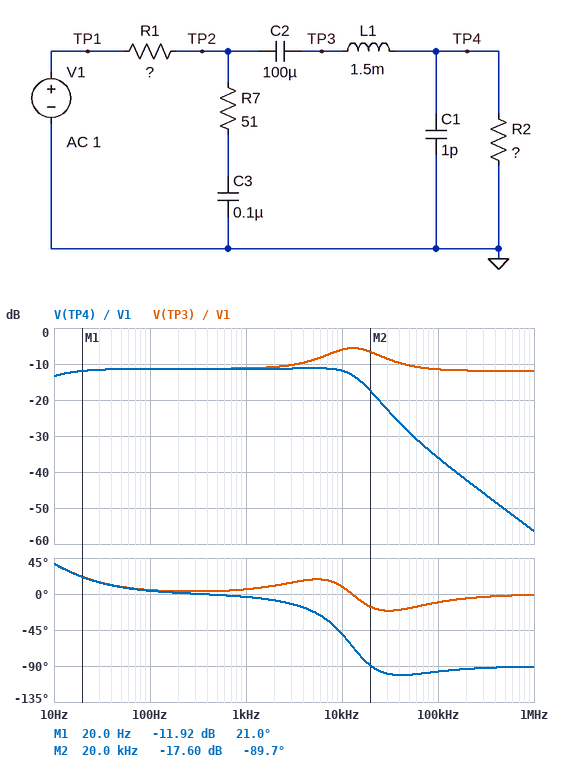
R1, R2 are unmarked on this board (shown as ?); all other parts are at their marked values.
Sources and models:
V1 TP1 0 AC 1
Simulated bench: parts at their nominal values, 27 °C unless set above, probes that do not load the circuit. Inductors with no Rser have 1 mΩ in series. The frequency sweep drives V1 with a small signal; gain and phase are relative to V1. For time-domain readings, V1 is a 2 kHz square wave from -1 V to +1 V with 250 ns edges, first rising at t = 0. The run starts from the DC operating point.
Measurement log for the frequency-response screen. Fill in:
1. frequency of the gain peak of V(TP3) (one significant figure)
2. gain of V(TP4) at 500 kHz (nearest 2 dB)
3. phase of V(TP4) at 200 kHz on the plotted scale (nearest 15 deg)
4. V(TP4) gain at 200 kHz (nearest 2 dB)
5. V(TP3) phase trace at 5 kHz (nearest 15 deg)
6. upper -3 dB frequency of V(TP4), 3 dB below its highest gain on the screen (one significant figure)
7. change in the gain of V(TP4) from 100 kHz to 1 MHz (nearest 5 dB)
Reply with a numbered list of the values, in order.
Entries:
1. 10 kHz
2. -50 dB
3. -90 deg
4. -42 dB
5. 15 deg
6. 10 kHz
7. -20 dB
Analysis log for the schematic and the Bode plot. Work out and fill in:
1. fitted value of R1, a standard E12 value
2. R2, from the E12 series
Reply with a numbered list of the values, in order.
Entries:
1. 150 Ω
2. 56 Ω
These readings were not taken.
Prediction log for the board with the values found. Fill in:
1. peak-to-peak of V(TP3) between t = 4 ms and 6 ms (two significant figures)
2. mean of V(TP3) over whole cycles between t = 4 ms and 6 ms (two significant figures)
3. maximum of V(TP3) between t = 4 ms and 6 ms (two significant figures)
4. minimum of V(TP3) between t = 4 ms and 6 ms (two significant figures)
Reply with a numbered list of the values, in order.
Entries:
1. 1.2 V
2. 210 mV
3. 820 mV
4. -390 mV
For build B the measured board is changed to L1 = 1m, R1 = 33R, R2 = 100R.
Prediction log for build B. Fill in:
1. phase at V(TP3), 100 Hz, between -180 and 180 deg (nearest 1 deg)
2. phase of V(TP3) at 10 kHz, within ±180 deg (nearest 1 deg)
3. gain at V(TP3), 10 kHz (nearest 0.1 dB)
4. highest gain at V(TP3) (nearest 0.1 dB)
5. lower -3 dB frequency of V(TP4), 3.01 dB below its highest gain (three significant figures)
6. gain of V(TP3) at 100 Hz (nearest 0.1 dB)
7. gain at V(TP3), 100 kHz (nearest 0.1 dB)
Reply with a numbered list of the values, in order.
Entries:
1. 7 deg
2. -2 deg
3. -2.3 dB
4. -2.2 dB
5. 12.0 Hz
6. -2.5 dB
7. -4.1 dB
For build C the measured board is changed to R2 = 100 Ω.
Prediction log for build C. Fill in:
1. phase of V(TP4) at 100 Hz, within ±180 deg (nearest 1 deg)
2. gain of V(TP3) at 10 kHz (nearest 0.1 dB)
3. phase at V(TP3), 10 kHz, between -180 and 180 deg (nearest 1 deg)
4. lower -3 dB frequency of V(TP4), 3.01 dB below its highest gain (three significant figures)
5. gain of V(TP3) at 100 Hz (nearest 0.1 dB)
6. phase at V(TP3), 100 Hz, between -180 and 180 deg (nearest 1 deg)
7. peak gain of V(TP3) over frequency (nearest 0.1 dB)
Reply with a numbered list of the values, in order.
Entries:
1. 3 deg
2. -6.3 dB
3. -3 deg
4. 6.36 Hz
5. -8.0 dB
6. 4 deg
7. -6.2 dB
